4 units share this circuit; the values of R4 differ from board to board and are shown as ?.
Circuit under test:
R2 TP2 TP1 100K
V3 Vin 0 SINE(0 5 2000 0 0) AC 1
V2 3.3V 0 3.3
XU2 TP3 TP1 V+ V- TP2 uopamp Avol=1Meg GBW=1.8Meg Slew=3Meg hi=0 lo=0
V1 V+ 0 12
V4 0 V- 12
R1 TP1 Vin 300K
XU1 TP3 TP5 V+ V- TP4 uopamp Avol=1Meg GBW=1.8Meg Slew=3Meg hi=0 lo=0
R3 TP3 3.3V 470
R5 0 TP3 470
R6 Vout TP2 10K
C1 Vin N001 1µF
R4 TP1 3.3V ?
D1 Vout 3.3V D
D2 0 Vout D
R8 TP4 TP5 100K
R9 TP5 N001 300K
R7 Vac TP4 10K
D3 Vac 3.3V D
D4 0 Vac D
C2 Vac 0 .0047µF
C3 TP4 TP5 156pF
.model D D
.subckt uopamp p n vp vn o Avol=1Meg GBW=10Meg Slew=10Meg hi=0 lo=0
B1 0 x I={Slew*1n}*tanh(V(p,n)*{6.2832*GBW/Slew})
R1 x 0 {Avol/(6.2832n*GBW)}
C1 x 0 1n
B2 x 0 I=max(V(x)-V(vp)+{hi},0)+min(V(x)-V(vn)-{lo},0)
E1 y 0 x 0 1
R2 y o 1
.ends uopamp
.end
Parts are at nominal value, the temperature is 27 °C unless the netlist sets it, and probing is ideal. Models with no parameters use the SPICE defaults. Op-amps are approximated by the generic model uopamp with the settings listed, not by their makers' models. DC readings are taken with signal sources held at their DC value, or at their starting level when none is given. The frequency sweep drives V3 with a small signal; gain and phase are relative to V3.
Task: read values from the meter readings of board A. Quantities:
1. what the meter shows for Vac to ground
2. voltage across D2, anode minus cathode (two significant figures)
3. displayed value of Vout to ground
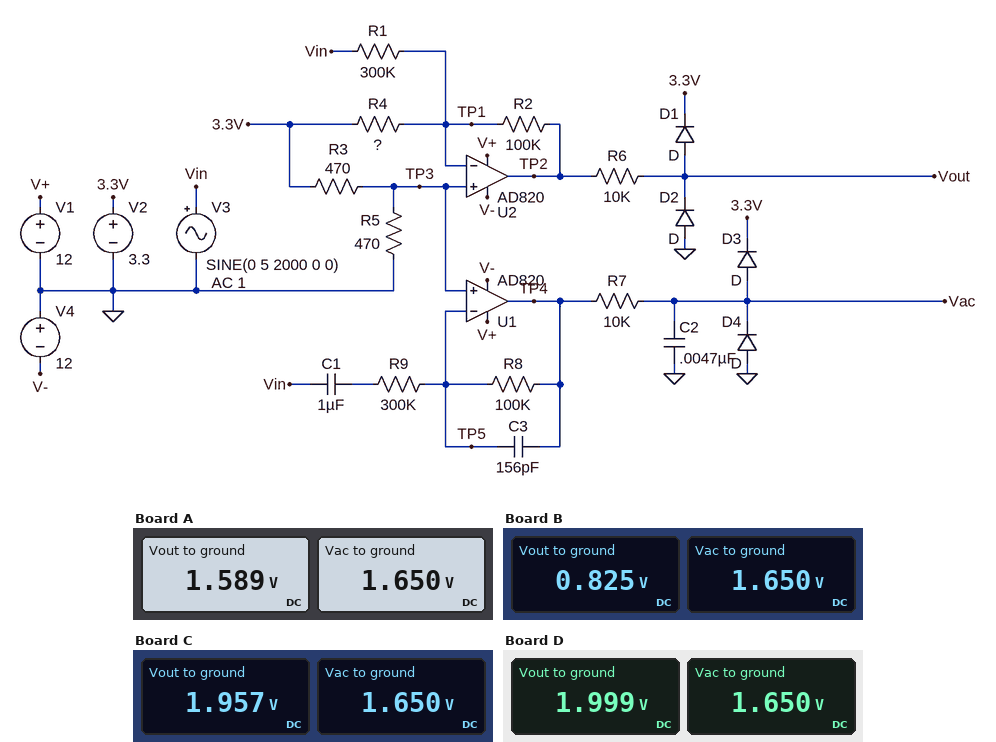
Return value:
1.650 V
-1.6 V
1.589 V
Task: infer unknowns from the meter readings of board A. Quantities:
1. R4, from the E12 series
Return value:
270 kΩ
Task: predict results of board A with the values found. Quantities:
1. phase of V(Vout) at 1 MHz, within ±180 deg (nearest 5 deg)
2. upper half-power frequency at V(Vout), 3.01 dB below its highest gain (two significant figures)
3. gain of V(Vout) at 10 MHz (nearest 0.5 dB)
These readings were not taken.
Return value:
135 deg
1.1 MHz
-29.0 dB
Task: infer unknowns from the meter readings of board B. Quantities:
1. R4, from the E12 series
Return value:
120 kΩ
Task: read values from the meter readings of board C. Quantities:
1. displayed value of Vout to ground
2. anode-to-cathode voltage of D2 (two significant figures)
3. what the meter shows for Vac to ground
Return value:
1.957 V
-2.0 V
1.650 V
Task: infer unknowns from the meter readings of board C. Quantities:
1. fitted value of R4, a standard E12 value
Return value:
680 kΩ
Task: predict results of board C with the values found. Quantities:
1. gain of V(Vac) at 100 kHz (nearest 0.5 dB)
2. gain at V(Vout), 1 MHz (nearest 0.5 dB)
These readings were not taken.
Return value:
-59.0 dB
-12.0 dB
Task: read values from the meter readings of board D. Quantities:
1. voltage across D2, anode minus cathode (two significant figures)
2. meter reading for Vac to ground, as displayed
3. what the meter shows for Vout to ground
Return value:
-2.0 V
1.650 V
1.999 V
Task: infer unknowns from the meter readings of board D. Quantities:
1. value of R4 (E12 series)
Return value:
820 kΩ
